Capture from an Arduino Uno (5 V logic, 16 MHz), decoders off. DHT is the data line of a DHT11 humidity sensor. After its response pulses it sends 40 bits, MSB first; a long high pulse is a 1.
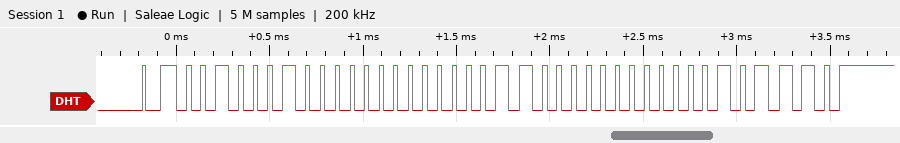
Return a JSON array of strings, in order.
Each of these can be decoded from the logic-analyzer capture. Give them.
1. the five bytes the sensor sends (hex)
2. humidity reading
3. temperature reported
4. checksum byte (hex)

["22 00 0C 00 2E", "34 %", "12.0 °C", "0x2E"]
